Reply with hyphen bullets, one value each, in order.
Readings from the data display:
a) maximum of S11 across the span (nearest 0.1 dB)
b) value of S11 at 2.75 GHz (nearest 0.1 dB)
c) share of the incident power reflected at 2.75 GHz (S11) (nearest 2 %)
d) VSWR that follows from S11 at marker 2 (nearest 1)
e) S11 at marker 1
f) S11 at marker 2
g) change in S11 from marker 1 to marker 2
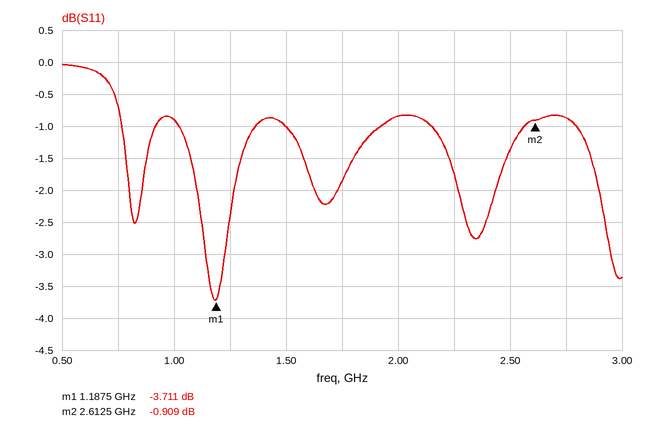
- 0.0 dB
- -0.9 dB
- 82 %
- 19
- -3.711 dB
- -0.909 dB
- 2.802 dB
